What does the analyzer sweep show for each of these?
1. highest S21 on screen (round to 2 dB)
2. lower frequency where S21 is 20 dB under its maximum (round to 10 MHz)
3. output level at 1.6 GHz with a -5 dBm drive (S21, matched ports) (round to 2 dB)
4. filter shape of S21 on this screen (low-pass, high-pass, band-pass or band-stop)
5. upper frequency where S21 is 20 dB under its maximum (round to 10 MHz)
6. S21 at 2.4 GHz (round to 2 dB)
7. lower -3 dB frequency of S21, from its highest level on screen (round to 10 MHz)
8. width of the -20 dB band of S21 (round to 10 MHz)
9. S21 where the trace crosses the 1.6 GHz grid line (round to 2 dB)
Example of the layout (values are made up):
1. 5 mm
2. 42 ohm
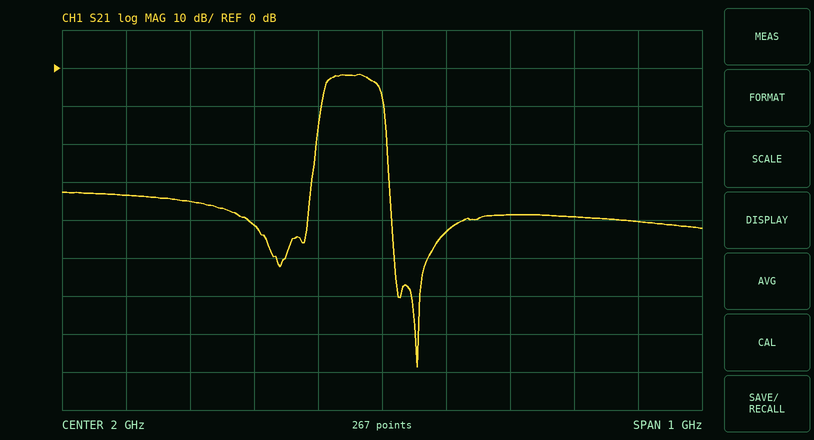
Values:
1. -2 dB
2. 1.90 GHz
3. -38 dBm
4. band-pass
5. 2.01 GHz
6. -40 dB
7. 1.91 GHz
8. 110 MHz
9. -34 dB
